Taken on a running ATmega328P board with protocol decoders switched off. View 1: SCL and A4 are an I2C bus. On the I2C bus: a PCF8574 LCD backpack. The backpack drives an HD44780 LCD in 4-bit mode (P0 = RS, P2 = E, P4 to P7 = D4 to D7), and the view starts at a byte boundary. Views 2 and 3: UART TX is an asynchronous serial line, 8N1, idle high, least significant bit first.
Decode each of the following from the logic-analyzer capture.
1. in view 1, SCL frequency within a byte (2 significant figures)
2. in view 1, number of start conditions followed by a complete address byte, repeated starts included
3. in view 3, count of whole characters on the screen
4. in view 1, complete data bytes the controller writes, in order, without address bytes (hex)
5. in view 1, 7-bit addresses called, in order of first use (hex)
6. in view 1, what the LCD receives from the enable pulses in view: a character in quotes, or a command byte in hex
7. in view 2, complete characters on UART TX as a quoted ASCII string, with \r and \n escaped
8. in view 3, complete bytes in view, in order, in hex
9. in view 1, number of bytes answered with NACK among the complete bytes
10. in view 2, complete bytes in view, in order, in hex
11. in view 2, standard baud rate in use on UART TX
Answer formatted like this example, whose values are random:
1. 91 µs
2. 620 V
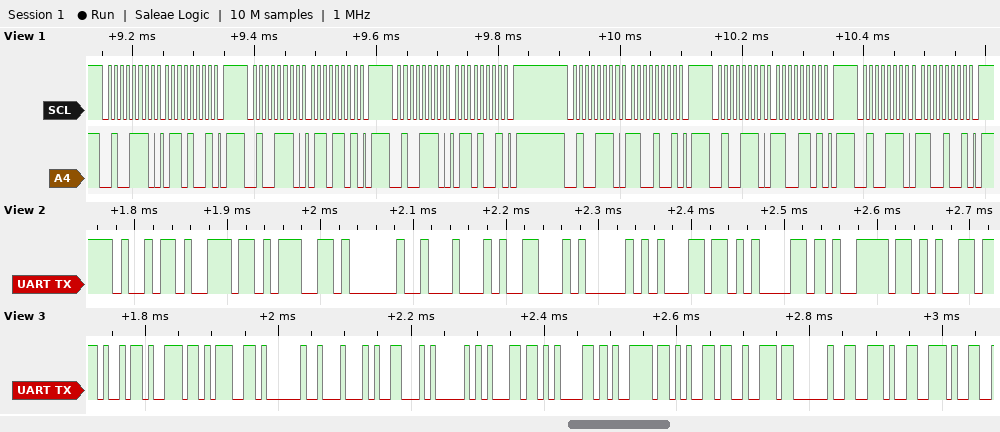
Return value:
1. 100 kHz
2. 6
3. 15
4. 69 6D 69 C9 CD C9
5. 0x27
6. 'l'
7. "ing DFPlaye"
8. 0x69 0x6E 0x67 0x20 0x44 0x46 0x50 0x6C 0x61 0x79 0x65 0x72 0x20 0x2E 0x2E
9. 0
10. 69 6E 67 20 44 46 50 6C 61 79 65
11. 115200 baud
